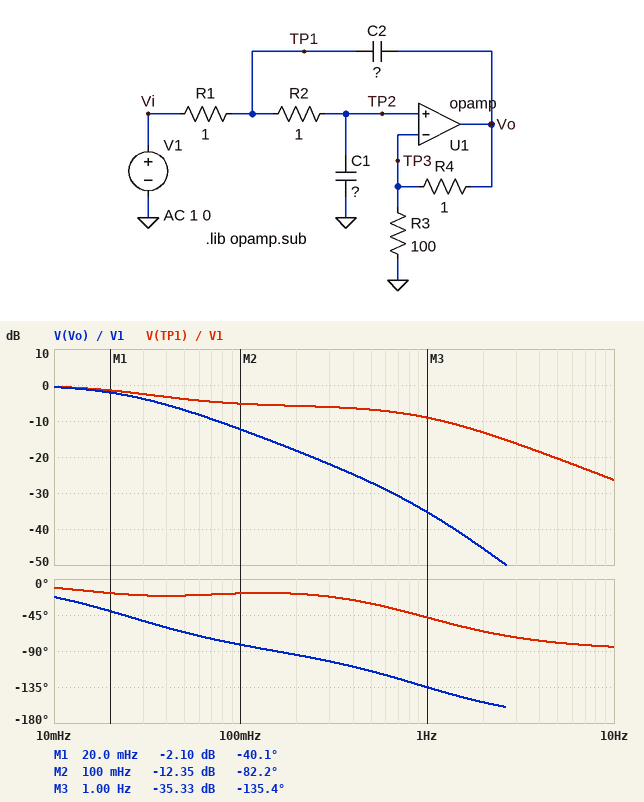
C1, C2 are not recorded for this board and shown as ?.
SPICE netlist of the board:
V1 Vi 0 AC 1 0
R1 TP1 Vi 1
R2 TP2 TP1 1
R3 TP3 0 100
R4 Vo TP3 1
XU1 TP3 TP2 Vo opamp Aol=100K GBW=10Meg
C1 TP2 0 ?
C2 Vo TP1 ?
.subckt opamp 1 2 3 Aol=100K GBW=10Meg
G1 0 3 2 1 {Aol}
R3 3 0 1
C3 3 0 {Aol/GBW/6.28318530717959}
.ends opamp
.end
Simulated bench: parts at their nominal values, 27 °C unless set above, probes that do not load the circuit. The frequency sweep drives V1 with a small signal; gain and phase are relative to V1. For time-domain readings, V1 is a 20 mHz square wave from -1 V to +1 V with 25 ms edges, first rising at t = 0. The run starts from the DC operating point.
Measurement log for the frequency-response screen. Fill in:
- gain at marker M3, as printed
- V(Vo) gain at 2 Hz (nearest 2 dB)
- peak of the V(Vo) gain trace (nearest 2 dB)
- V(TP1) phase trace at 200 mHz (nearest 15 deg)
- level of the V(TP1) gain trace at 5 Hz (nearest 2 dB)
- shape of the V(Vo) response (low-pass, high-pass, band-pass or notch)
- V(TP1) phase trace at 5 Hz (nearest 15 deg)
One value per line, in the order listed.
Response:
-35.33 dB
-46 dB
0 dB
-15 deg
-20 dB
low-pass
-75 deg
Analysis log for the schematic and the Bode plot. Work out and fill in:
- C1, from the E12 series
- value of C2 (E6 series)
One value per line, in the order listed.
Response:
3.3 F
330 mF
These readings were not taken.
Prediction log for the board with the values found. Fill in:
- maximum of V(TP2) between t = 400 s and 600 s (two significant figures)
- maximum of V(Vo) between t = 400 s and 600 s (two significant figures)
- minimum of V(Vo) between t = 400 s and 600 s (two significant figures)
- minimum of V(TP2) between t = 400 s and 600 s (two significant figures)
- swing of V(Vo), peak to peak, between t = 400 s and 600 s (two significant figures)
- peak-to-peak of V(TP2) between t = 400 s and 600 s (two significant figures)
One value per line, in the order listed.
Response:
960 mV
970 mV
-970 mV
-960 mV
1.9 V
1.9 V
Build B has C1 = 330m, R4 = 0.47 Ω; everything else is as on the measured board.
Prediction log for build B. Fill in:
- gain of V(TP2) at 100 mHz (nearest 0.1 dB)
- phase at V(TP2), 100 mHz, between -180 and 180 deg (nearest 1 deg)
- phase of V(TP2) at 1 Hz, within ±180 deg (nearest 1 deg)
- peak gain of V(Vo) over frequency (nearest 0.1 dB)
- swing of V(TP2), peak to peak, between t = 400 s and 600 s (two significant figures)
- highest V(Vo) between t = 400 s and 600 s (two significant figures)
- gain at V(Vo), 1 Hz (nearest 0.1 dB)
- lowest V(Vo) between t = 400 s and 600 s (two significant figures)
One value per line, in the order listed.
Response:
-0.4 dB
-23 deg
-129 deg
0 dB
2.0 V
1.0 V
-14.4 dB
-1.0 V
